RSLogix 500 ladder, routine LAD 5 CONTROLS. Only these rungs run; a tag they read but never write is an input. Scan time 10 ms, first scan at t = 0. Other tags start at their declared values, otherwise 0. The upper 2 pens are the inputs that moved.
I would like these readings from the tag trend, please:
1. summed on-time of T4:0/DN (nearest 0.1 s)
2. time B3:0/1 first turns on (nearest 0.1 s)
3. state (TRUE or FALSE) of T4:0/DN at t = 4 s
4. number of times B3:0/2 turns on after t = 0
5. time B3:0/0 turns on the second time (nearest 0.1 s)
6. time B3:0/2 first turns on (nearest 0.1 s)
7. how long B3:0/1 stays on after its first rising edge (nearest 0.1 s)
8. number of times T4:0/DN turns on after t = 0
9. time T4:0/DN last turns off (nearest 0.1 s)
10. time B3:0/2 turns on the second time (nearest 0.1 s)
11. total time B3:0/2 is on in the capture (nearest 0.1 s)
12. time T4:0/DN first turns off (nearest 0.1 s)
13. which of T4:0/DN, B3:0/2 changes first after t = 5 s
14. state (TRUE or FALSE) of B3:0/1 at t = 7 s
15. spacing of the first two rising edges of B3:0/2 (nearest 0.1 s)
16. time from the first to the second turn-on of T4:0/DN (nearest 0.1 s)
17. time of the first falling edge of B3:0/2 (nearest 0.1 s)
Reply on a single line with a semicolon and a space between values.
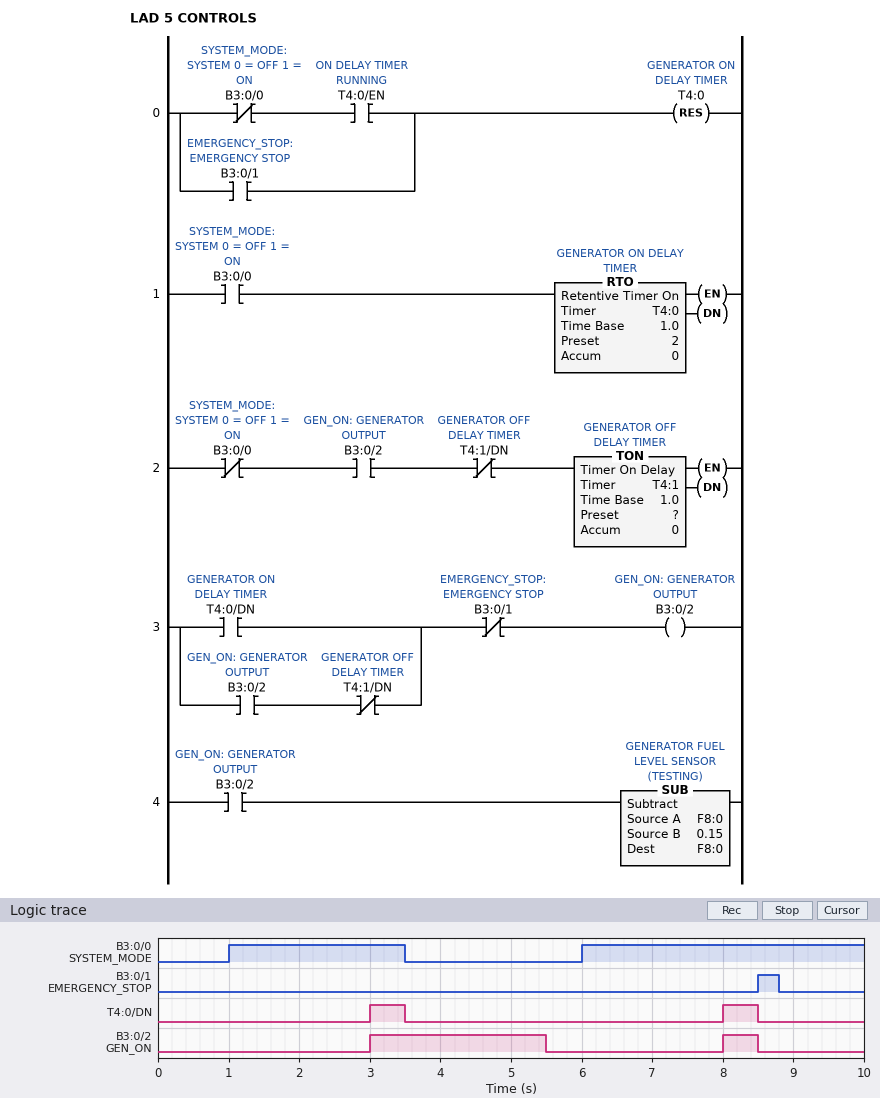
1.0 s; 8.5 s; FALSE; 2; 6.0 s; 3.0 s; 0.3 s; 2; 8.5 s; 8.0 s; 3.0 s; 3.5 s; B3:0/2; FALSE; 5.0 s; 5.0 s; 5.5 s
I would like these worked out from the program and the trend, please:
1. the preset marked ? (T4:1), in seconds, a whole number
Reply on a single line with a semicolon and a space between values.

2 s
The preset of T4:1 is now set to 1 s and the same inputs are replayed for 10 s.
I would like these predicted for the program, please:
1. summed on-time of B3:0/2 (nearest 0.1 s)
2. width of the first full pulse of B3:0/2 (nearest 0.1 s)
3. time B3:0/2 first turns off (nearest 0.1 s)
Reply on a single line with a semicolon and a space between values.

2.0 s; 1.5 s; 4.5 s
